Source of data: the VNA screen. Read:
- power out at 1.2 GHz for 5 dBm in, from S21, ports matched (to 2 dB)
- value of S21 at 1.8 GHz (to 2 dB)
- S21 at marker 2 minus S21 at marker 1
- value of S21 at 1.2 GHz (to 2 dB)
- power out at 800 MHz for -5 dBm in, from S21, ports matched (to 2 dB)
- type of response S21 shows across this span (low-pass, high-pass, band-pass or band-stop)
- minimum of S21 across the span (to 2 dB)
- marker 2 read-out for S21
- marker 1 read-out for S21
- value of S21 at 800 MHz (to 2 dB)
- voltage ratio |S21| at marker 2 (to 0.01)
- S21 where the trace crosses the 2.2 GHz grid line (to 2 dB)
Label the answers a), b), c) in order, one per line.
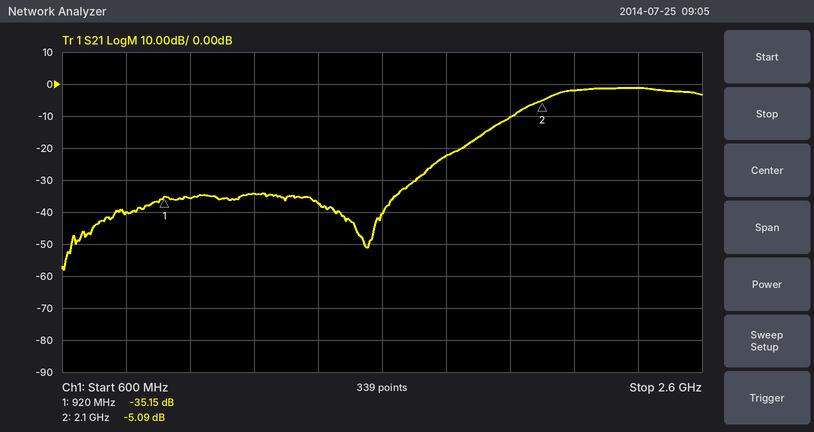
a) -30 dBm
b) -22 dB
c) 30.06 dB
d) -34 dB
e) -46 dBm
f) high-pass
g) -58 dB
h) -5.09 dB
i) -35.15 dB
j) -40 dB
k) 0.56
l) -2 dB
